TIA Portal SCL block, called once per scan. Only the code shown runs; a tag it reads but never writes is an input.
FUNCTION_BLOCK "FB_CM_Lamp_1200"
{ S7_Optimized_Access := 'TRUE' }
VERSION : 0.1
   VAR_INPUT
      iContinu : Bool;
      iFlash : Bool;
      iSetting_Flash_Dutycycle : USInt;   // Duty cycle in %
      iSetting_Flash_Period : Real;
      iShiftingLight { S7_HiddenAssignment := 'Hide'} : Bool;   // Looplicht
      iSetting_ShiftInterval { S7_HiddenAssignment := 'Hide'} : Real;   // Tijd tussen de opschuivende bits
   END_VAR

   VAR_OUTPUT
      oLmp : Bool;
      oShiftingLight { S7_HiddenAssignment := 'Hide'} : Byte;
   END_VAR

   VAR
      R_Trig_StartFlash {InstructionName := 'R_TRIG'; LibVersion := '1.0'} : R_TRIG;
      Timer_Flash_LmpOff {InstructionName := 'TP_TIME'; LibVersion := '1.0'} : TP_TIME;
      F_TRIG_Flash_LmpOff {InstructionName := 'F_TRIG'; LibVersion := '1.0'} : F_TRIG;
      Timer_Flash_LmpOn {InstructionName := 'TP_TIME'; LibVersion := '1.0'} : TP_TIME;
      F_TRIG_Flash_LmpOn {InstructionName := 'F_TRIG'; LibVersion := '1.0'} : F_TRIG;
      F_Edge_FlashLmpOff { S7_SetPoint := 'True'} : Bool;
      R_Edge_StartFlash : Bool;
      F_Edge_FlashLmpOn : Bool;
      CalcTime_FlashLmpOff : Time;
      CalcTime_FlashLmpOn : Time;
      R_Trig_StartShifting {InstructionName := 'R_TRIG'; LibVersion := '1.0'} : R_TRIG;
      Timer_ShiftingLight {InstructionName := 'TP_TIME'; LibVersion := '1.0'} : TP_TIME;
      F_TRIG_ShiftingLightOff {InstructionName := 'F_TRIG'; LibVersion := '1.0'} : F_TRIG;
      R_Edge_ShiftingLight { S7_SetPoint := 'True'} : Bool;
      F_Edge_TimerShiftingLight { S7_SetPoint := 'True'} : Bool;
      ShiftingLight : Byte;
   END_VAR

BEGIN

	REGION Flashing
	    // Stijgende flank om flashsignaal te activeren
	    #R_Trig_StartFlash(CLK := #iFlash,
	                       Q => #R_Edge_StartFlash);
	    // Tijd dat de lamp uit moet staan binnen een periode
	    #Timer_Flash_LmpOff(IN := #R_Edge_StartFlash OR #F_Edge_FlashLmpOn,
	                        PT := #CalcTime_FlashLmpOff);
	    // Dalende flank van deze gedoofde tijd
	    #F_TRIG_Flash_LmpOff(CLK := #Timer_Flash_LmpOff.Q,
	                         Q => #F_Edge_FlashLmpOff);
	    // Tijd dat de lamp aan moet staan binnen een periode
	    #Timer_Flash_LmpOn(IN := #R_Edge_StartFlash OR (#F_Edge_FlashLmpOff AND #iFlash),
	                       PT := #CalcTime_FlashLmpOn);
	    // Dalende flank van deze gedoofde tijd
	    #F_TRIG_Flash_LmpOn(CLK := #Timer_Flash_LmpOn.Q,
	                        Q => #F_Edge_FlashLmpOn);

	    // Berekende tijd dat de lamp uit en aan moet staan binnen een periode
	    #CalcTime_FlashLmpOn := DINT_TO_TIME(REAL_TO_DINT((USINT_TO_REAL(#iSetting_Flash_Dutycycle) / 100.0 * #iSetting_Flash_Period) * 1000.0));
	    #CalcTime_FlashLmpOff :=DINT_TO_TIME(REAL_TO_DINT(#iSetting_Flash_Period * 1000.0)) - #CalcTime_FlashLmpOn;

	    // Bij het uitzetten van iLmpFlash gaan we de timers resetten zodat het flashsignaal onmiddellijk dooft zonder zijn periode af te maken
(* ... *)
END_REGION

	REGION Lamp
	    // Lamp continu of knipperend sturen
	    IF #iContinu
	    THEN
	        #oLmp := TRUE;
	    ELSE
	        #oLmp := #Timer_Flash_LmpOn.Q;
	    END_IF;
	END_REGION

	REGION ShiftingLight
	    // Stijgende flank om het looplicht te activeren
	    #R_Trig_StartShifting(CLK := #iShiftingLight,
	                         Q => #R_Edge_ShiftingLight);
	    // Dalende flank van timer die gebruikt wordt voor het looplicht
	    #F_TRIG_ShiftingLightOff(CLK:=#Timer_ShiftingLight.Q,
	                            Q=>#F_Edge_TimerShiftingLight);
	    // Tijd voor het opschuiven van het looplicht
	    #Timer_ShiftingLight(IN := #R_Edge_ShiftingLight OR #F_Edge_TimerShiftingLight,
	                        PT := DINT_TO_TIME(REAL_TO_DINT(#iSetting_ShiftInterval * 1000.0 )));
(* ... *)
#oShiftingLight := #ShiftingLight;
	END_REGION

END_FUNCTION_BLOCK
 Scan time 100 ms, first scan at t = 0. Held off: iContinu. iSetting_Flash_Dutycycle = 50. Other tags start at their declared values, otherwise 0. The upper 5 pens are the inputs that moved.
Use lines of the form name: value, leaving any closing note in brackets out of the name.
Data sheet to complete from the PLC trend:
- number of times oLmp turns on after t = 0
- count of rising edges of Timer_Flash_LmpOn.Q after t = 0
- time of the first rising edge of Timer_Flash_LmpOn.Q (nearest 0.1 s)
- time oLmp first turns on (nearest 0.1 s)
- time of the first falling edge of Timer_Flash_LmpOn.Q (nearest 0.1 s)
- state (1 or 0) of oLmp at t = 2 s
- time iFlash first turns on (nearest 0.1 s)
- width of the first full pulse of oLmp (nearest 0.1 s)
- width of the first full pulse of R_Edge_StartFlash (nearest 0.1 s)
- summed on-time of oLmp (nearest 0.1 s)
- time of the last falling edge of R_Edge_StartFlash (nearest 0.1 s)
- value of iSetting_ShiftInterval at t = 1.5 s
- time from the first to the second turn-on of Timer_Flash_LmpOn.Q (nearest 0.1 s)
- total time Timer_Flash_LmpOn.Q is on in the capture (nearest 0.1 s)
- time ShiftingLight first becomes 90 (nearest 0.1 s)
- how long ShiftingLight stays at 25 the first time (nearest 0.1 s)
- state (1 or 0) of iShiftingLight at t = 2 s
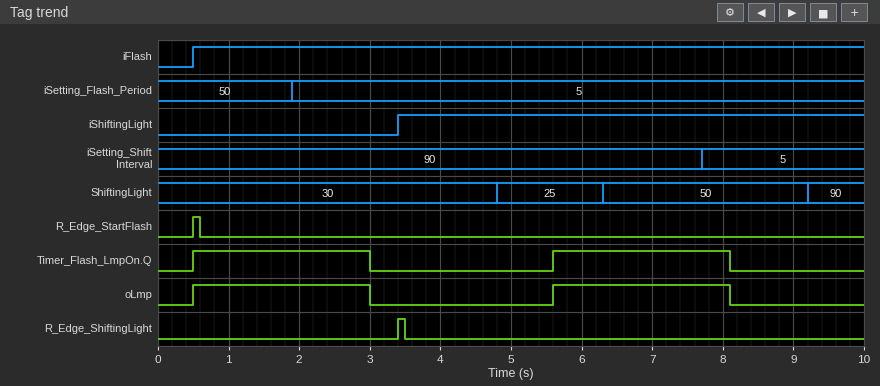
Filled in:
number of times oLmp turns on after t = 0: 2
count of rising edges of Timer_Flash_LmpOn.Q after t = 0: 2
time of the first rising edge of Timer_Flash_LmpOn.Q: 0.5 s
time oLmp first turns on: 0.5 s
time of the first falling edge of Timer_Flash_LmpOn.Q: 3.0 s
state (1 or 0) of oLmp at t = 2 s: 1
time iFlash first turns on: 0.5 s
width of the first full pulse of oLmp: 2.5 s
width of the first full pulse of R_Edge_StartFlash: 0.1 s
summed on-time of oLmp: 5.0 s
time of the last falling edge of R_Edge_StartFlash: 0.6 s
value of iSetting_ShiftInterval at t = 1.5 s: 90
time from the first to the second turn-on of Timer_Flash_LmpOn.Q: 5.1 s
total time Timer_Flash_LmpOn.Q is on in the capture: 5.0 s
time ShiftingLight first becomes 90: 9.2 s
how long ShiftingLight stays at 25 the first time: 1.5 s
state (1 or 0) of iShiftingLight at t = 2 s: 0
